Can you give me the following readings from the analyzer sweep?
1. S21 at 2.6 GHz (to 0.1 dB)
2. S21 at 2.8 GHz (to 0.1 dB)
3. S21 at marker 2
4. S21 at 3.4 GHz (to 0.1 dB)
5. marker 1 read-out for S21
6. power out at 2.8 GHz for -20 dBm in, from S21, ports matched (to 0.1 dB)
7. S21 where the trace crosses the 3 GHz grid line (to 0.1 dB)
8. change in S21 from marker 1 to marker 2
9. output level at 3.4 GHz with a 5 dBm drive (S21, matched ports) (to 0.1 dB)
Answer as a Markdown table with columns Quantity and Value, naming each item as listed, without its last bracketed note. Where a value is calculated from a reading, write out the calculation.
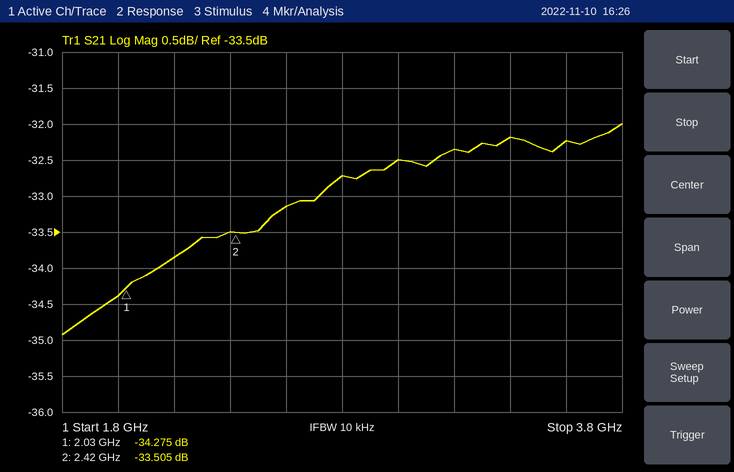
| Quantity | Value |
|---|---|
| S21 at 2.6 GHz | -33.1 dB |
| S21 at 2.8 GHz | -32.7 dB |
| S21 at marker 2 | -33.505 dB |
| S21 at 3.4 GHz | -32.2 dB |
| marker 1 read-out for S21 | -34.275 dB |
| power out at 2.8 GHz for -20 dBm in, from S21, ports matched | -20 dBm + (-32.7 dB) = -52.7 dBm |
| S21 where the trace crosses the 3 GHz grid line | -32.5 dB |
| change in S21 from marker 1 to marker 2 | -33.505 − (-34.275) = 0.770 dB |
| output level at 3.4 GHz with a 5 dBm drive (S21, matched ports) | 5 dBm + (-32.2 dB) = -27.2 dBm |
